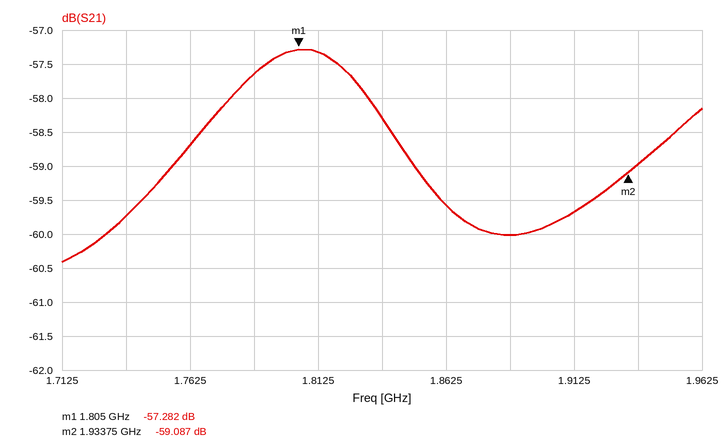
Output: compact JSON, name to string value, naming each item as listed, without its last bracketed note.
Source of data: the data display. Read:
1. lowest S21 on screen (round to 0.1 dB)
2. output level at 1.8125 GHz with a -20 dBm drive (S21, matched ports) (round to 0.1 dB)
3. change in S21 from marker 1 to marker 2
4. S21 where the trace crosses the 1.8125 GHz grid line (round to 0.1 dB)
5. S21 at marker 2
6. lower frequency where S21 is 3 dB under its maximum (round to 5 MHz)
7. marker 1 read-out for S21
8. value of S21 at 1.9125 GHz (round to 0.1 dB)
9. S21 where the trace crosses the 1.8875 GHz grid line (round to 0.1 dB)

{"lowest S21 on screen": "-60.4 dB", "output level at 1.8125 GHz with a -20 dBm drive (S21, matched ports)": "-77.3 dBm", "change in S21 from marker 1 to marker 2": "-1.805 dB", "S21 where the trace crosses the 1.8125 GHz grid line": "-57.3 dB", "S21 at marker 2": "-59.087 dB", "lower frequency where S21 is 3 dB under its maximum": "1.720 GHz", "marker 1 read-out for S21": "-57.282 dB", "value of S21 at 1.9125 GHz": "-59.7 dB", "S21 where the trace crosses the 1.8875 GHz grid line": "-60.0 dB"}
